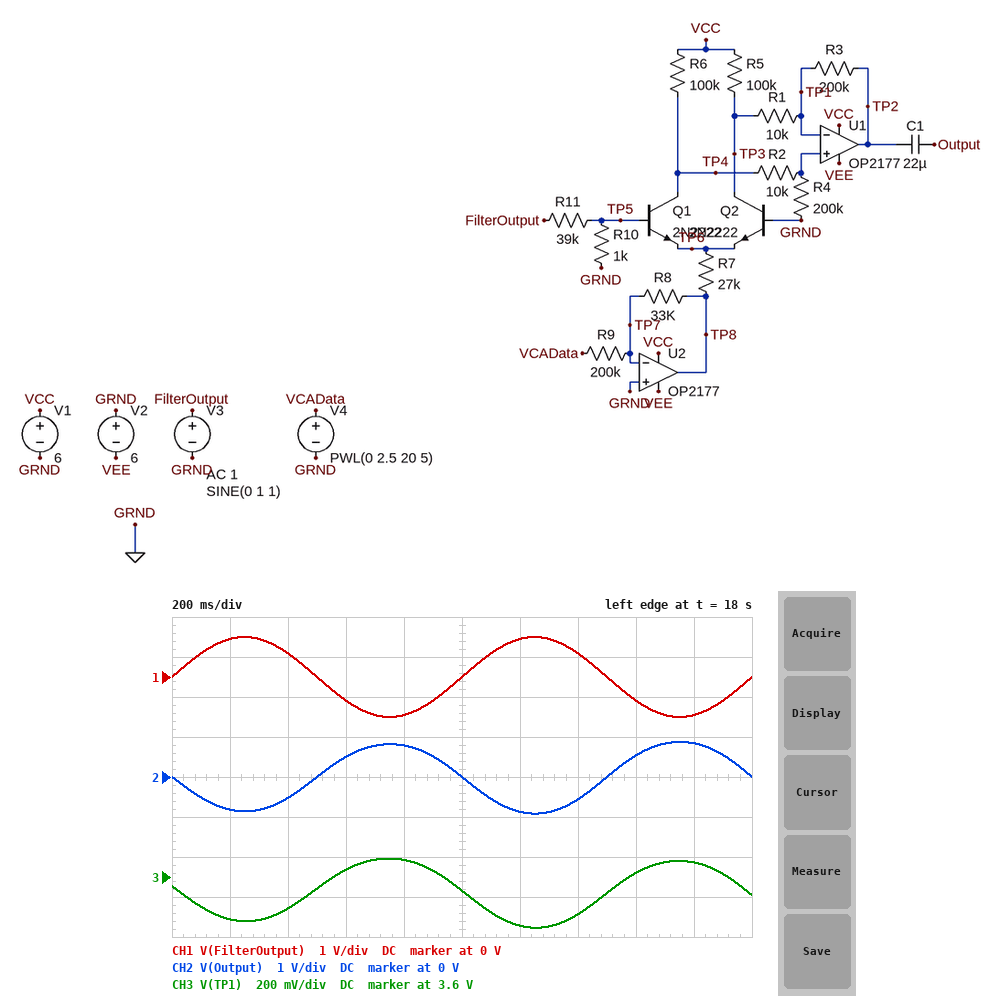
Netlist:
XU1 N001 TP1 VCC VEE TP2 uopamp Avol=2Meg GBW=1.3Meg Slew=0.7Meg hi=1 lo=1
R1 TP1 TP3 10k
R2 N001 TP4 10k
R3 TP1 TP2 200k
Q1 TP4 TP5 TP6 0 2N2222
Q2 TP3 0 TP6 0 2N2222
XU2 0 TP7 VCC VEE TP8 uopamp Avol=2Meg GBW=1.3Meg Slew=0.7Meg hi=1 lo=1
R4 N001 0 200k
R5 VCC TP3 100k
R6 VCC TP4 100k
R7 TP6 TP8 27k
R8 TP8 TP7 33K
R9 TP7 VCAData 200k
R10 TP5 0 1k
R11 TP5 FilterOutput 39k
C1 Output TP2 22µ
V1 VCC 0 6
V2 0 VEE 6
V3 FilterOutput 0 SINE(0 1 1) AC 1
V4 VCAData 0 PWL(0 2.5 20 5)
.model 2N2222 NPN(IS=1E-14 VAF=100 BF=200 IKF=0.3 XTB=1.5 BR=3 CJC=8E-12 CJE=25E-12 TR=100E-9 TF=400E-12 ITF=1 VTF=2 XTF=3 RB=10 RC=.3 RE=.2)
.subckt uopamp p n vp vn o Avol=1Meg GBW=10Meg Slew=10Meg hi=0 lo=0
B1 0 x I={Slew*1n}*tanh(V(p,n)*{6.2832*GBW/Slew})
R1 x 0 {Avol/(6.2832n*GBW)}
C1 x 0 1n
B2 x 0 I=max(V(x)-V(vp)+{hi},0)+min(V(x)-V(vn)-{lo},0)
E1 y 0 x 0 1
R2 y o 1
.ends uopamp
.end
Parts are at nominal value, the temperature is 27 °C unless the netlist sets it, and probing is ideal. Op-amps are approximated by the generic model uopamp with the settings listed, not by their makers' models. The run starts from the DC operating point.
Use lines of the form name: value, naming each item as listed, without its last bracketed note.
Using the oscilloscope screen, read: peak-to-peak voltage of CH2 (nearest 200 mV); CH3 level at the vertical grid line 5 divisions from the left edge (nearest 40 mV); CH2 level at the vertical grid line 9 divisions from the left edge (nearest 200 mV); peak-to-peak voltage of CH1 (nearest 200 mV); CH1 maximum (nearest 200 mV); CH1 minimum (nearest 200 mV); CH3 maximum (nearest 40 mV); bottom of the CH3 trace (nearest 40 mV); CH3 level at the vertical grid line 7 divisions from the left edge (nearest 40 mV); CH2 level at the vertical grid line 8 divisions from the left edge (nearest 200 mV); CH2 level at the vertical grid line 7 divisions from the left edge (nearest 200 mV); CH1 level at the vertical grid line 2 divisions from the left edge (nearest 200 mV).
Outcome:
peak-to-peak voltage of CH2: 1.8 V
CH3 level at the vertical grid line 5 divisions from the left edge: 3.52 V
CH2 level at the vertical grid line 9 divisions from the left edge: 800 mV
peak-to-peak voltage of CH1: 2.0 V
CH1 maximum: 1.0 V
CH1 minimum: -1.0 V
CH3 maximum: 3.68 V
bottom of the CH3 trace: 3.36 V
CH3 level at the vertical grid line 7 divisions from the left edge: 3.40 V
CH2 level at the vertical grid line 8 divisions from the left edge: 600 mV
CH2 level at the vertical grid line 7 divisions from the left edge: -600 mV
CH1 level at the vertical grid line 2 divisions from the left edge: 600 mV
